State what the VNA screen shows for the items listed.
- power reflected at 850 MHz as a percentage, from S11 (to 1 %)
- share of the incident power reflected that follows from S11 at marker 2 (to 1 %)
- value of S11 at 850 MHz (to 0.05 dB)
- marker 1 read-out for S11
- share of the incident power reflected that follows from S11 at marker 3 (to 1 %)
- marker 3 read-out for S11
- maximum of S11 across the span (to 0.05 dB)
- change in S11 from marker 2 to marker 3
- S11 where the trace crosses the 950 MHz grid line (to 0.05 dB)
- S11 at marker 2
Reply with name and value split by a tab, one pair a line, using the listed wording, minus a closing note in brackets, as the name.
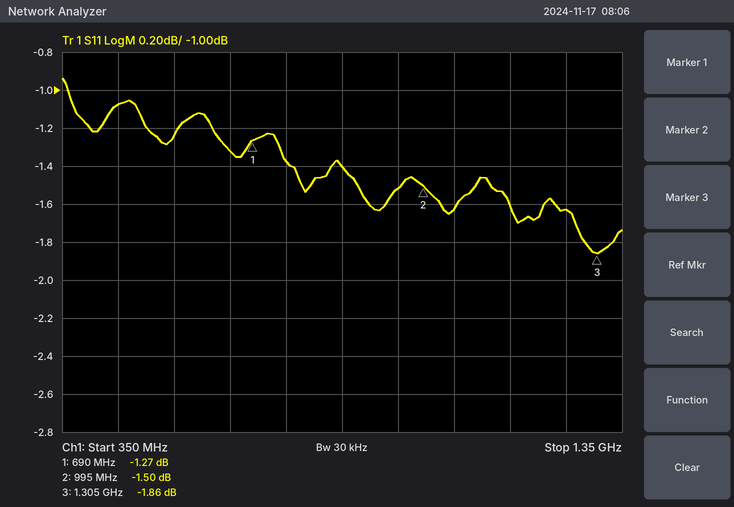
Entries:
power reflected at 850 MHz as a percentage, from S11	72 %
share of the incident power reflected that follows from S11 at marker 2	71 %
value of S11 at 850 MHz	-1.40 dB
marker 1 read-out for S11	-1.27 dB
share of the incident power reflected that follows from S11 at marker 3	65 %
marker 3 read-out for S11	-1.86 dB
maximum of S11 across the span	-0.95 dB
change in S11 from marker 2 to marker 3	-0.36 dB
S11 where the trace crosses the 950 MHz grid line	-1.50 dB
S11 at marker 2	-1.50 dB
